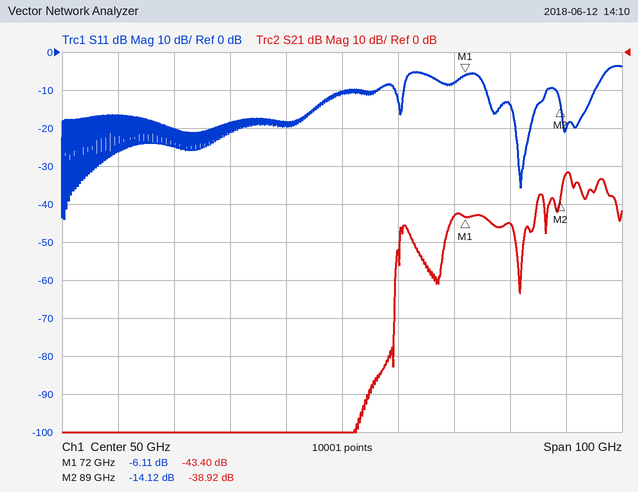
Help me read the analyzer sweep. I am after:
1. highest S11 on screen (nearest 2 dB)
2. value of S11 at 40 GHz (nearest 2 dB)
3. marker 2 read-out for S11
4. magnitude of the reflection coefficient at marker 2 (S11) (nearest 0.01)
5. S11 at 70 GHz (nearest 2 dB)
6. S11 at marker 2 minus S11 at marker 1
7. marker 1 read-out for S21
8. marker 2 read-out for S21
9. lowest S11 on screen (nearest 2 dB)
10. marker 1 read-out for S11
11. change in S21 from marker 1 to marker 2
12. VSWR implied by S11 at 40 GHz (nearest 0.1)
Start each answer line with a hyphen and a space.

- -4 dB
- -18 dB
- -14.12 dB
- 0.20
- -8 dB
- -8.01 dB
- -43.40 dB
- -38.92 dB
- -44 dB
- -6.11 dB
- 4.48 dB
- 1.3
